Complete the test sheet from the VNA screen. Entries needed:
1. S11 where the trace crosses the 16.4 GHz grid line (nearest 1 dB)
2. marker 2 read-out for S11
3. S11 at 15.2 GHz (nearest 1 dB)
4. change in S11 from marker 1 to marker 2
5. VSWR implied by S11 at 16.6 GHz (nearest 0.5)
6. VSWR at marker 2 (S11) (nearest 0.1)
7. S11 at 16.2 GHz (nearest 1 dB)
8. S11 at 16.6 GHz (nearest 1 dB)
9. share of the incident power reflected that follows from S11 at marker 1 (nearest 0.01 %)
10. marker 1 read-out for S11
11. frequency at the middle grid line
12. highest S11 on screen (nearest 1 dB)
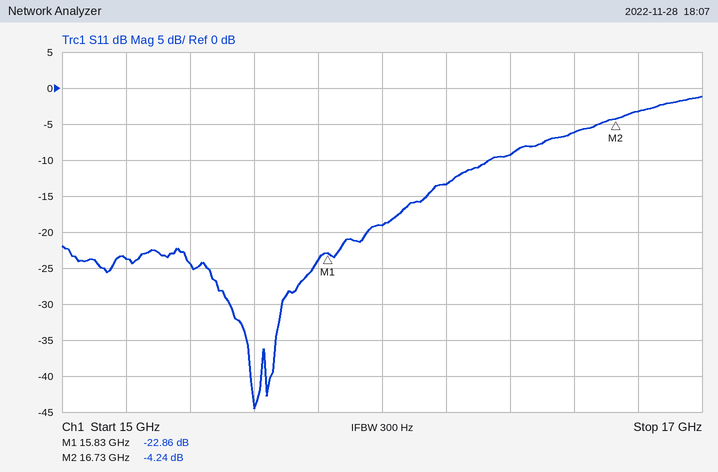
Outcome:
-9 dB
-4.24 dB
-24 dB
18.62 dB
3.0
4.2
-13 dB
-6 dB
0.52 %
-22.86 dB
16 GHz
-1 dB
